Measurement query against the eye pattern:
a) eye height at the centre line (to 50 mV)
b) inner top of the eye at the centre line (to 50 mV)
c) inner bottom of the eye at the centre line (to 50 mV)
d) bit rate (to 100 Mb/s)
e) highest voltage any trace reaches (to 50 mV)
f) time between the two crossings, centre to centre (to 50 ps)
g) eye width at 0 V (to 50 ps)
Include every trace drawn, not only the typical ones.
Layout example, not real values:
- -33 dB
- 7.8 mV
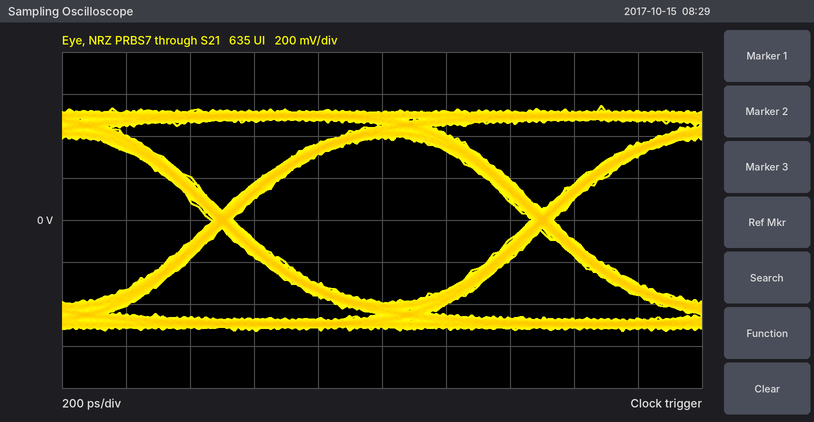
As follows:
- 800 mV
- 400 mV
- -400 mV
- 1.0 Gb/s
- 550 mV
- 1.00 ns
- 950 ps
